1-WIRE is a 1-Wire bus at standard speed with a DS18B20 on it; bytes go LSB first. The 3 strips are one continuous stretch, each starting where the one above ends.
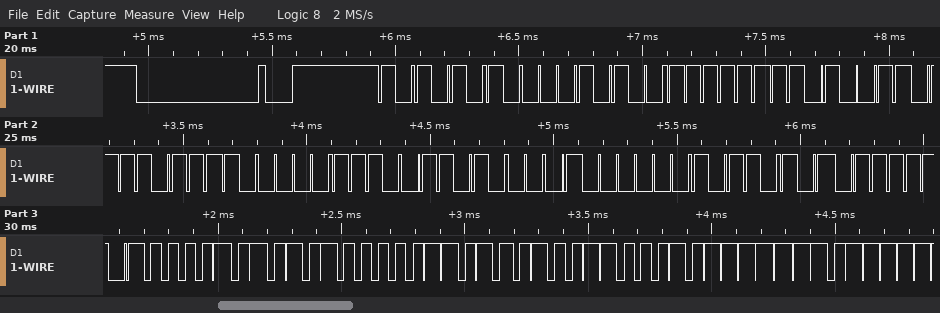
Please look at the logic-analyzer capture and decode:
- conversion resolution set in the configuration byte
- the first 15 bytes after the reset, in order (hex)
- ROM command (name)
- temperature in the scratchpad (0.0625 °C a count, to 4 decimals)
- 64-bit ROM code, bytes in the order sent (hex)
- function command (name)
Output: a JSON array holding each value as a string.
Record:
["12 bits", "55 28 FF B2 7B 70 16 02 AD BE 50 05 4B 46 7F", "Match ROM", "85.0000 °C", "28 FF B2 7B 70 16 02 AD", "Read Scratchpad"]
